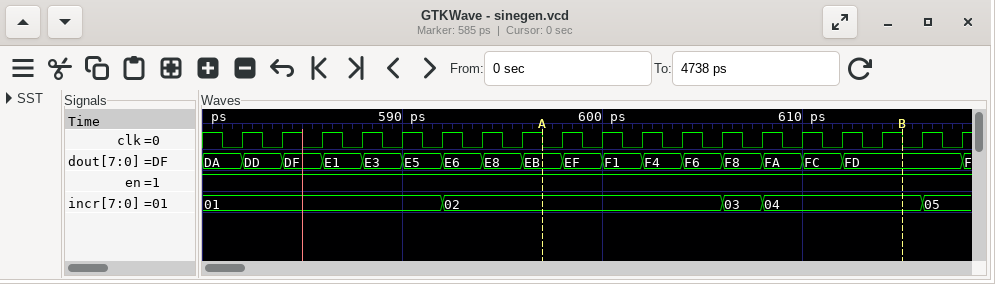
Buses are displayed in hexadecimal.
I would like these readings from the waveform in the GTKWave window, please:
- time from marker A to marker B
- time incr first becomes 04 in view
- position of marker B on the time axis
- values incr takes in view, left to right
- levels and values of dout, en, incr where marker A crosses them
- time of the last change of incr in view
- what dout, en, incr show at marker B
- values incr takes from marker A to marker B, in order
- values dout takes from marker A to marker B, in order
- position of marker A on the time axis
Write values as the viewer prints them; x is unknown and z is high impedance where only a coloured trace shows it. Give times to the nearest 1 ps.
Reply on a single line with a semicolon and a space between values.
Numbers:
18 ps; 608 ps; 615 ps; 01, 02, 03, 04, 05; dout=EB, en=1, incr=02; 616 ps; dout=FD, en=1, incr=04; 02, 03, 04; EB, EF, F1, F4, F6, F8, FA, FC, FD; 597 ps
